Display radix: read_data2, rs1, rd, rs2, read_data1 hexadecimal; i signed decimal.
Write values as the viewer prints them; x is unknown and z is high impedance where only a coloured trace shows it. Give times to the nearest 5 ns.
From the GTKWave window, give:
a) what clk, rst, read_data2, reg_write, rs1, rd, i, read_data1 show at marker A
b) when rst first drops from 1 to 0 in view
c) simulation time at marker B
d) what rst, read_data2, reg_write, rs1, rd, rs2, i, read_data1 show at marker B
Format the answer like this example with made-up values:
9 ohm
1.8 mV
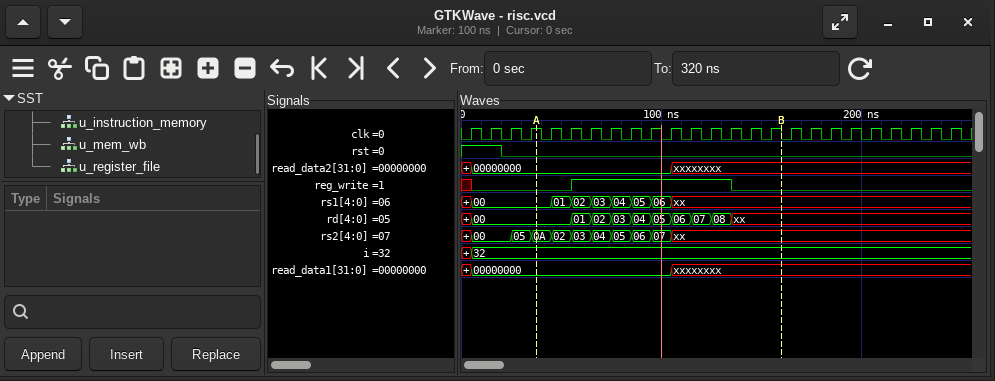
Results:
clk=1, rst=0, read_data2=00000000, reg_write=0, rs1=00, rd=00, i=32, read_data1=00000000
20 ns
160 ns
rst=0, read_data2=xxxxxxxx, reg_write=0, rs1=xx, rd=xx, rs2=xx, i=32, read_data1=xxxxxxxx
